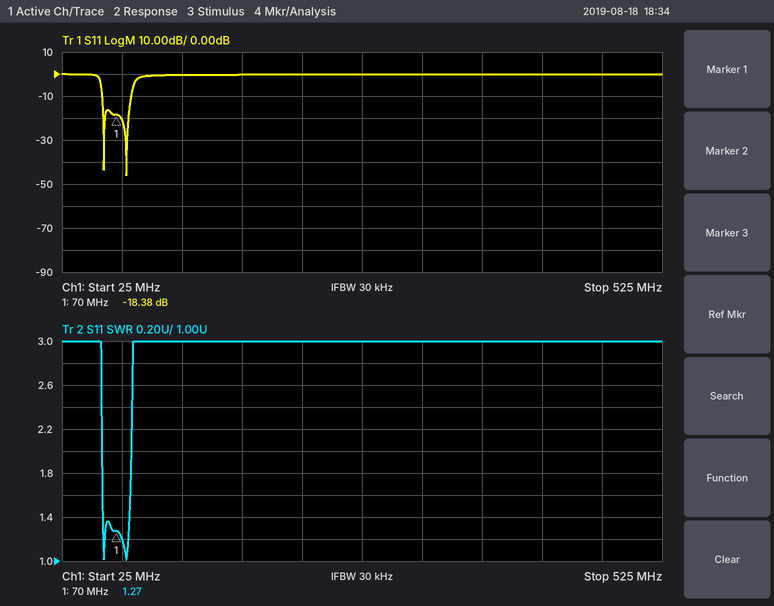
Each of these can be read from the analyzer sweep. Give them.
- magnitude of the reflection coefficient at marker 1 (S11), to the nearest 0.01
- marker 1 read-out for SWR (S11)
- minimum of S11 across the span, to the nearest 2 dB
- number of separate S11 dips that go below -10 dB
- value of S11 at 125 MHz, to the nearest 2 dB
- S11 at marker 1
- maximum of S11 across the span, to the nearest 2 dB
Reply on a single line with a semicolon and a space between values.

0.12; 1.27; -46 dB; 2; 0 dB; -18.38 dB; 0 dB
